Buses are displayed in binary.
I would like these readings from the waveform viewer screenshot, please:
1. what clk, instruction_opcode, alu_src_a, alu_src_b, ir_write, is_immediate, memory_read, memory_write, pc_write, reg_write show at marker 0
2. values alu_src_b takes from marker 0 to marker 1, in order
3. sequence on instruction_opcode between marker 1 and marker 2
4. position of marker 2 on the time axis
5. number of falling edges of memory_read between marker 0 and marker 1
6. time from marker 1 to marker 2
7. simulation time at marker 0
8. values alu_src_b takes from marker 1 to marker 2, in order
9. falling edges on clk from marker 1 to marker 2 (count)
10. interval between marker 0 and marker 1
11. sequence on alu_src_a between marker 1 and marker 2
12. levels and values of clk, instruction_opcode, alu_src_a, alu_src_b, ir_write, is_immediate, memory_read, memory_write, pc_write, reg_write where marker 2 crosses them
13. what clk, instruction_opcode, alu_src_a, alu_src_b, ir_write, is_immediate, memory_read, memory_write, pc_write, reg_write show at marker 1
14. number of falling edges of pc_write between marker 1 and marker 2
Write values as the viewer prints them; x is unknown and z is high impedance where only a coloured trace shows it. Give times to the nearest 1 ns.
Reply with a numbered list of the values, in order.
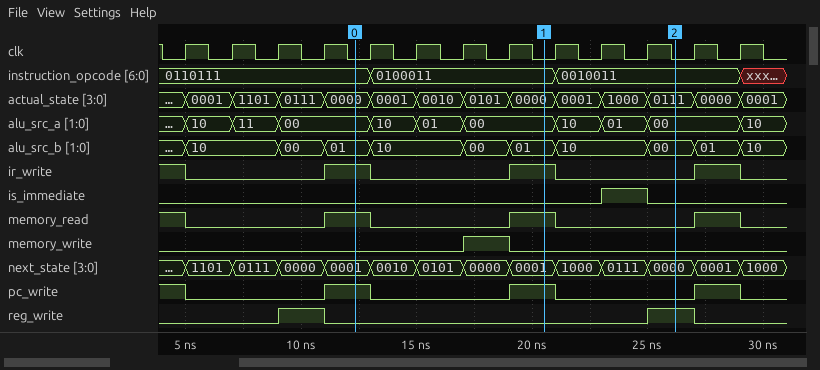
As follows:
1. clk=0, instruction_opcode=0110111, alu_src_a=00, alu_src_b=01, ir_write=1, is_immediate=0, memory_read=1, memory_write=0, pc_write=1, reg_write=0
2. 01, 10, 00, 01
3. 0100011, 0010011
4. 26 ns
5. 1
6. 6 ns
7. 12 ns
8. 01, 10, 00
9. 3
10. 8 ns
11. 00, 10, 01, 00
12. clk=0, instruction_opcode=0010011, alu_src_a=00, alu_src_b=00, ir_write=0, is_immediate=0, memory_read=0, memory_write=0, pc_write=0, reg_write=1
13. clk=0, instruction_opcode=0100011, alu_src_a=00, alu_src_b=01, ir_write=1, is_immediate=0, memory_read=1, memory_write=0, pc_write=1, reg_write=0
14. 1
